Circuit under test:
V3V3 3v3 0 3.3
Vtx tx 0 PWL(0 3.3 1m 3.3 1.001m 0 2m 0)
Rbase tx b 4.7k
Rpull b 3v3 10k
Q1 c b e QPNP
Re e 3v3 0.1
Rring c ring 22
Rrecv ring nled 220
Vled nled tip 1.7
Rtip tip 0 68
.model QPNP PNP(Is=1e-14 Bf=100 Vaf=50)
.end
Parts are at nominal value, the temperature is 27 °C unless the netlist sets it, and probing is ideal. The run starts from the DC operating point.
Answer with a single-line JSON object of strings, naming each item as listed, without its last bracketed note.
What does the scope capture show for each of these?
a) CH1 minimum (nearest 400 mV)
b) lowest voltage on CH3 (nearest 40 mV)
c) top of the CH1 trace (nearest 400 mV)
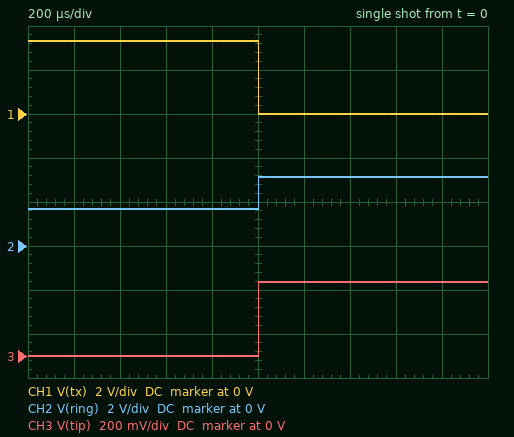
{"CH1 minimum": "0 V", "lowest voltage on CH3": "0 V", "top of the CH1 trace": "3.2 V"}
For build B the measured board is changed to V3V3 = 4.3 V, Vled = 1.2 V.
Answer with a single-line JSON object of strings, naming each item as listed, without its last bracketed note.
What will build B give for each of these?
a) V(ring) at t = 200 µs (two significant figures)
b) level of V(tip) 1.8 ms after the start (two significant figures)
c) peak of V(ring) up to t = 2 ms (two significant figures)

{"V(ring) at t = 200 µs": "1.5 V", "level of V(tip) 1.8 ms after the start": "660 mV", "peak of V(ring) up to t = 2 ms": "4.0 V"}
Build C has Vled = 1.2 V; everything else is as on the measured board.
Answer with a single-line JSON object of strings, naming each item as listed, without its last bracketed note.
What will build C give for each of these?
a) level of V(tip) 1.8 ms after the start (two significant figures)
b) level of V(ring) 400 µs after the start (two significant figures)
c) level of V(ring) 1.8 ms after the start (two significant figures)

{"level of V(tip) 1.8 ms after the start": "440 mV", "level of V(ring) 400 µs after the start": "1.2 V", "level of V(ring) 1.8 ms after the start": "3.1 V"}
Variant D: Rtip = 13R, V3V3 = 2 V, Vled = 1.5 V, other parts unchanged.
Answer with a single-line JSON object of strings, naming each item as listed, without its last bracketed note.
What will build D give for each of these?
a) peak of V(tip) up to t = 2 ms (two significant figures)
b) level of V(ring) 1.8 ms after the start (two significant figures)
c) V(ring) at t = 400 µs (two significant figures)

{"peak of V(tip) up to t = 2 ms": "22 mV", "level of V(ring) 1.8 ms after the start": "1.9 V", "V(ring) at t = 400 µs": "1.5 V"}
